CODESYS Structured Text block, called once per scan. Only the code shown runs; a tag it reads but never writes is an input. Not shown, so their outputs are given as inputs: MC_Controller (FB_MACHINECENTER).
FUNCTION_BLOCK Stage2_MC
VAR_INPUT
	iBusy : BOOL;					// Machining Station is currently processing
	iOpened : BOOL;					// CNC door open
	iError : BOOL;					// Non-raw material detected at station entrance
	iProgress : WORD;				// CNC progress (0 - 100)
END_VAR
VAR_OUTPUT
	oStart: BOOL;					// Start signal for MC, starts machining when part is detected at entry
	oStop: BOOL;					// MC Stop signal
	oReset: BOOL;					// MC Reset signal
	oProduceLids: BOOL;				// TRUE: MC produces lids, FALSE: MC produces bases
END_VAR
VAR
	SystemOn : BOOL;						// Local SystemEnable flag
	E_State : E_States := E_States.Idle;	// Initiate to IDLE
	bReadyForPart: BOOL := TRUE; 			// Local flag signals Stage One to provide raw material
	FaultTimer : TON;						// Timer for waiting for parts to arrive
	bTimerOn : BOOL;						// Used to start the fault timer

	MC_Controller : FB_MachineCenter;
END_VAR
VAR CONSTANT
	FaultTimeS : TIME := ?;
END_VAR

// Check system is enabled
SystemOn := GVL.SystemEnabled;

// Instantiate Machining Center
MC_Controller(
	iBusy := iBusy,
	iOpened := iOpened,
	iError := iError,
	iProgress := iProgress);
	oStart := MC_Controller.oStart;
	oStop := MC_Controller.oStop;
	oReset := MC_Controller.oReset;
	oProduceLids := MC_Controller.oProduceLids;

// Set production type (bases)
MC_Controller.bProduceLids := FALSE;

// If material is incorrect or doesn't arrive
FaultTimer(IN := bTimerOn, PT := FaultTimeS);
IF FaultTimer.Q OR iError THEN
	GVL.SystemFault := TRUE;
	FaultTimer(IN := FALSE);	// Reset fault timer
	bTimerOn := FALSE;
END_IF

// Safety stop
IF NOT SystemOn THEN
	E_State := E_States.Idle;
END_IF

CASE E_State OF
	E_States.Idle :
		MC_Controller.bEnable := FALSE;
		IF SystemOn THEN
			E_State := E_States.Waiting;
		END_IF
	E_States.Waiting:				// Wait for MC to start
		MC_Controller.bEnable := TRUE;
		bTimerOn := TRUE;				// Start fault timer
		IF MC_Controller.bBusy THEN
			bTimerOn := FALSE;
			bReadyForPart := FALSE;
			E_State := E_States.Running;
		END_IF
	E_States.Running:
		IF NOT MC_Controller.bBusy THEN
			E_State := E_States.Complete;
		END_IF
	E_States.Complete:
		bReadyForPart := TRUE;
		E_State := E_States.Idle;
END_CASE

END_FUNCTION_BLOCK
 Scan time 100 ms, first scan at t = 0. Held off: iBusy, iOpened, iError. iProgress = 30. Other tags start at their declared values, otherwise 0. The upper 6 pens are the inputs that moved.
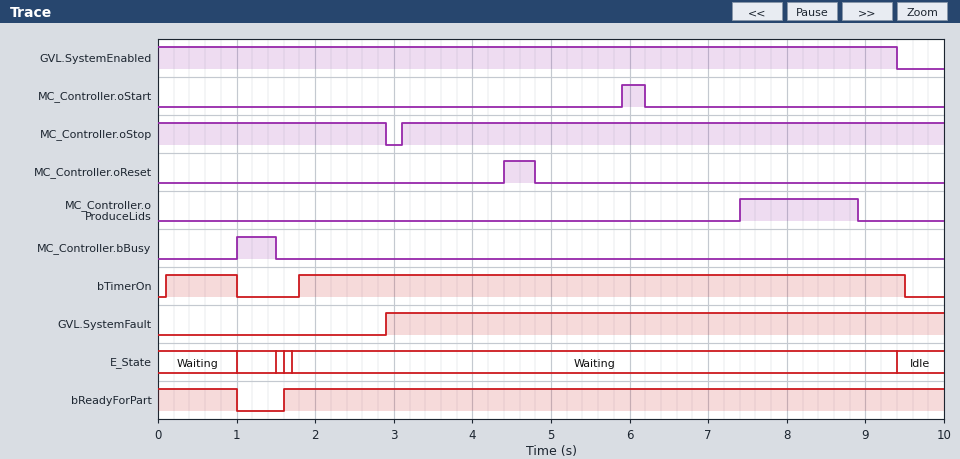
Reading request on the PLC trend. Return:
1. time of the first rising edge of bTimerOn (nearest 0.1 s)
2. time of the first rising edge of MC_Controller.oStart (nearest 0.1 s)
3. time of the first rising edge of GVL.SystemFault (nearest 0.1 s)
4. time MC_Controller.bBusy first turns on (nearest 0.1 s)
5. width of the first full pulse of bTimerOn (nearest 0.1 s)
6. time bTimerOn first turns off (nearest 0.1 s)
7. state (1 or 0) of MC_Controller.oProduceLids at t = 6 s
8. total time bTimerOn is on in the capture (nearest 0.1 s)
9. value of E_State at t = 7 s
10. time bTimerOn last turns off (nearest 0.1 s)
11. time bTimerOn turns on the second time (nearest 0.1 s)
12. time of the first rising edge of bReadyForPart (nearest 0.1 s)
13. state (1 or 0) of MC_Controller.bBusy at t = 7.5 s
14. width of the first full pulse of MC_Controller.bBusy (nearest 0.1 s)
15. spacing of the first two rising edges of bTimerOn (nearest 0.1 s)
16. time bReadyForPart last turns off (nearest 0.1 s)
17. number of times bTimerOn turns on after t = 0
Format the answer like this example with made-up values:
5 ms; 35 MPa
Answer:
0.1 s; 5.9 s; 2.9 s; 1.0 s; 0.9 s; 1.0 s; 0; 8.6 s; Waiting; 9.5 s; 1.8 s; 1.6 s; 0; 0.5 s; 1.7 s; 1.0 s; 2
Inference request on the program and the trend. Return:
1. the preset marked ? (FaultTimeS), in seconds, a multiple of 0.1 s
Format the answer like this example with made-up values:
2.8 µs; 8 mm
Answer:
1.0 s
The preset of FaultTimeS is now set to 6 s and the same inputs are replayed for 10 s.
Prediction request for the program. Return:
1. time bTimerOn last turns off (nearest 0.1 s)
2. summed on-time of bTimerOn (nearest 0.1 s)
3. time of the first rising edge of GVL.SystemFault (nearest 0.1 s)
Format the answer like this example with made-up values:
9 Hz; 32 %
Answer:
1.0 s; 9.1 s; 7.9 s
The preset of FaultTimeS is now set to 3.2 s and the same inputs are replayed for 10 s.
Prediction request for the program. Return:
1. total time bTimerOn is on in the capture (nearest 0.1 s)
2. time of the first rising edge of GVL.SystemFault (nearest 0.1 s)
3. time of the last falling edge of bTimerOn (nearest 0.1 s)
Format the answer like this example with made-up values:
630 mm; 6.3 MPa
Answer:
9.1 s; 5.1 s; 1.0 s
